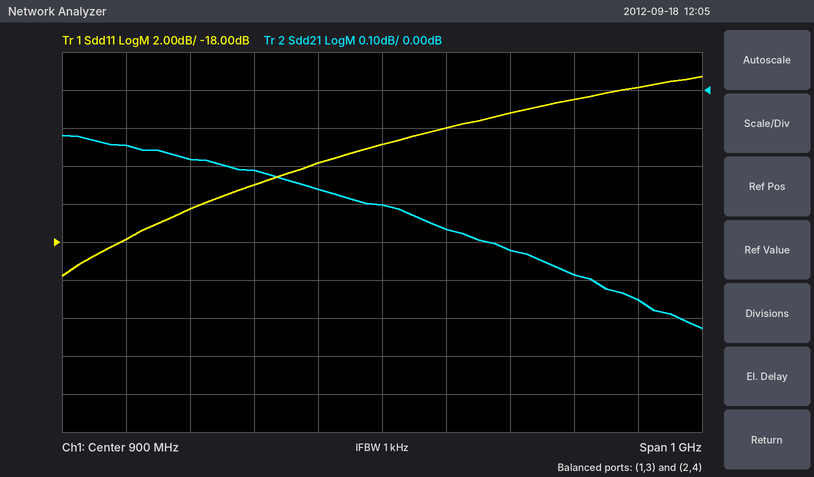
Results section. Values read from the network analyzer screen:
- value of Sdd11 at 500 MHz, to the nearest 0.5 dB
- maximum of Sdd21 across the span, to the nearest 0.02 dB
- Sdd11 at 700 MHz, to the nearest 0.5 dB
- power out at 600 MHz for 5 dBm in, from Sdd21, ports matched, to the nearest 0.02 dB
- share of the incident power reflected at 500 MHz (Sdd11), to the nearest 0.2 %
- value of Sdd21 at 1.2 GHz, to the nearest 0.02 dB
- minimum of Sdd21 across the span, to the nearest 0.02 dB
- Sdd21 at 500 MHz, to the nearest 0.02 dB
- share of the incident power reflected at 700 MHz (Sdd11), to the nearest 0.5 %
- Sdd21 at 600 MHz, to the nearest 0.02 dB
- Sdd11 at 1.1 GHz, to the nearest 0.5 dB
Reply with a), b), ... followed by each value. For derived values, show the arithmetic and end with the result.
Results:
a) -18.0 dB
b) -0.12 dB
c) -15.0 dB
d) 5 dBm + (-0.18 dB) = 4.82 dBm
e) 10^(-18/10) ≈ 1.6 %
f) -0.48 dB
g) -0.62 dB
h) -0.14 dB
i) 10^(-15/10) ≈ 3.16 %, so 3.0 % to the nearest 0.5 %
j) -0.18 dB
k) -11.0 dB
